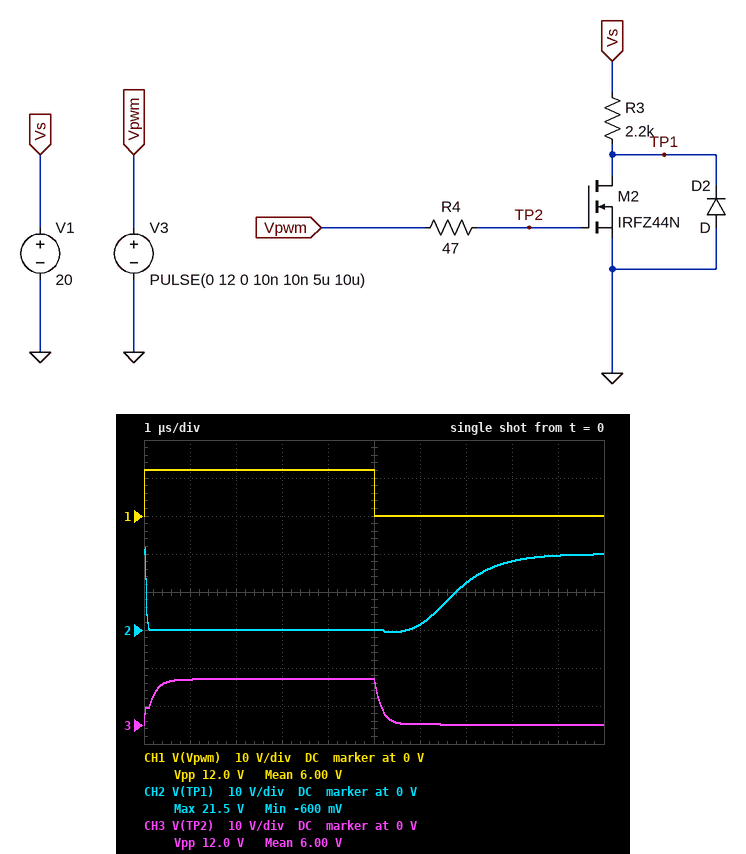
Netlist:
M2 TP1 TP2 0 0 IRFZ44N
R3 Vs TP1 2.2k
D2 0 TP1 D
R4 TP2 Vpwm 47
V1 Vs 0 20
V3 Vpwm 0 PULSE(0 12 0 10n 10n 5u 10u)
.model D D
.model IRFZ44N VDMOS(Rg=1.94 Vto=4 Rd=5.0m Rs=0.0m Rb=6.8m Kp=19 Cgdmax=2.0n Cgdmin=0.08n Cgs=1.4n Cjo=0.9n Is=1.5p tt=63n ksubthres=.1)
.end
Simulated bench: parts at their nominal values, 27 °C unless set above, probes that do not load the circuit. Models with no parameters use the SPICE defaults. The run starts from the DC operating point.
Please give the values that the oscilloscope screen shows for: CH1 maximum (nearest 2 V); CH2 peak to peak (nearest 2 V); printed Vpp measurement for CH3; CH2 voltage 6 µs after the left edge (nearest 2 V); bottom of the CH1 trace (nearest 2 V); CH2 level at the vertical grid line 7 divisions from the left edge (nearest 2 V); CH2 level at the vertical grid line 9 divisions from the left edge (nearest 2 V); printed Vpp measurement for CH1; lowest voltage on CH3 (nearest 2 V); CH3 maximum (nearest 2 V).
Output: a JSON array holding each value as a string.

["12 V", "22 V", "12.0 V", "2 V", "0 V", "12 V", "20 V", "12.0 V", "0 V", "12 V"]
